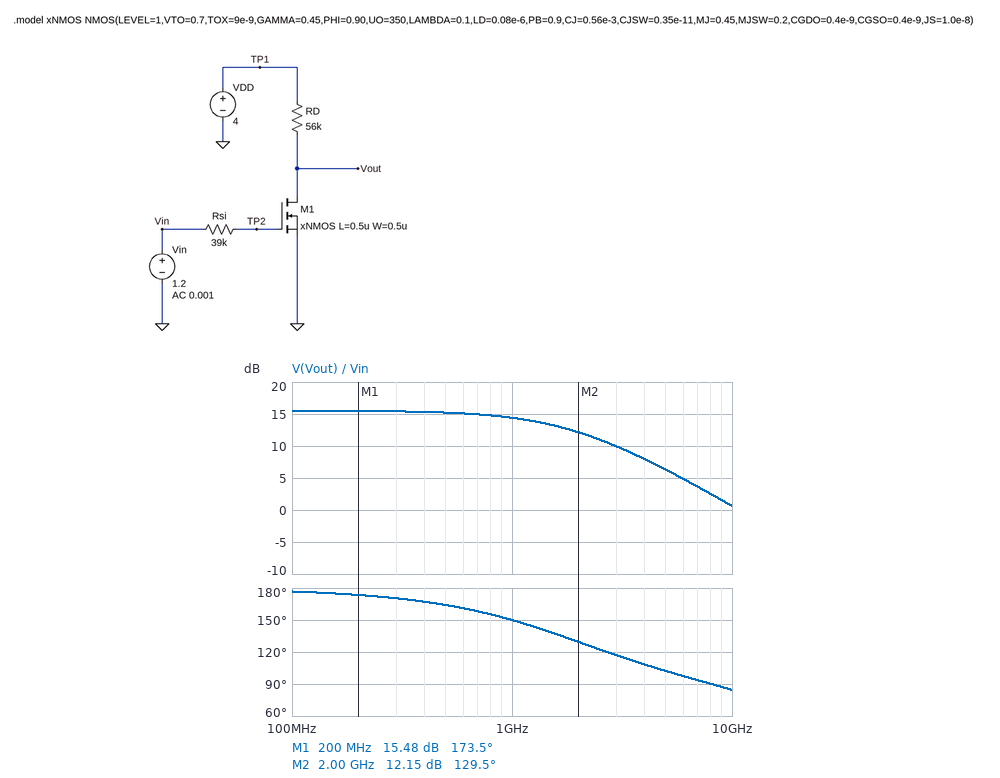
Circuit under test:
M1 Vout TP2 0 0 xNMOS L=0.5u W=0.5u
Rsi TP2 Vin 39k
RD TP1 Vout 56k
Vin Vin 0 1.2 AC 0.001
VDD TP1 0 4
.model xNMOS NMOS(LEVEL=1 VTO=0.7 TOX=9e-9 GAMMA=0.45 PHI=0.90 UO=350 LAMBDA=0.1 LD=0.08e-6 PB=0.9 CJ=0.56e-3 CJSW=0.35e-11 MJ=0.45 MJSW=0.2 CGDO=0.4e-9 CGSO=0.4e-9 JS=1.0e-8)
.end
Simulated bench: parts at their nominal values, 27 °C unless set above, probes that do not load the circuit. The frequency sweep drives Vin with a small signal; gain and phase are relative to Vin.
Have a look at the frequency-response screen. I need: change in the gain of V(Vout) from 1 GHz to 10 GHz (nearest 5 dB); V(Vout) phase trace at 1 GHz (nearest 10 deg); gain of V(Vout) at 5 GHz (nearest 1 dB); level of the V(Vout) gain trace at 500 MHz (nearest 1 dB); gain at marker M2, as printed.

-15 dB
150 deg
6 dB
15 dB
12.15 dB
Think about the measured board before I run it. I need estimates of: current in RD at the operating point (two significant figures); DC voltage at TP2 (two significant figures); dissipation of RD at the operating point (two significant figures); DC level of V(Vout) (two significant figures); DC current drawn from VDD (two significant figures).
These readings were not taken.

30 µA
1.2 V
52 µW
2.3 V
30 µA
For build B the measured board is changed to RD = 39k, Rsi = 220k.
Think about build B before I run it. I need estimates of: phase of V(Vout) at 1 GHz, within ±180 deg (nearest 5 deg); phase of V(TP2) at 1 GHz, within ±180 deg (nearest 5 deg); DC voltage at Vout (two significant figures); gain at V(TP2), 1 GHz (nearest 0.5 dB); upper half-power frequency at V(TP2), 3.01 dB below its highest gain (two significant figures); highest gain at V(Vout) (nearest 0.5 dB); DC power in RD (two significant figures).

110 deg
-65 deg
2.8 V
-8.5 dB
410 MHz
13.0 dB
39 µW
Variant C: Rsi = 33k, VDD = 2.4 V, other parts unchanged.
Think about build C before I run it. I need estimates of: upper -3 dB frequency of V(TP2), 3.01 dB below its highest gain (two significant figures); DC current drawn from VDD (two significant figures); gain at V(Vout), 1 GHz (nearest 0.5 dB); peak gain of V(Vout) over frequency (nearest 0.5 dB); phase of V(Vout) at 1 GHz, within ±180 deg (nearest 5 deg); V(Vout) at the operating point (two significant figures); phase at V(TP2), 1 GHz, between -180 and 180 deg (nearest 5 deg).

2.3 GHz
27 µA
13.5 dB
14.5 dB
155 deg
890 mV
-20 deg
